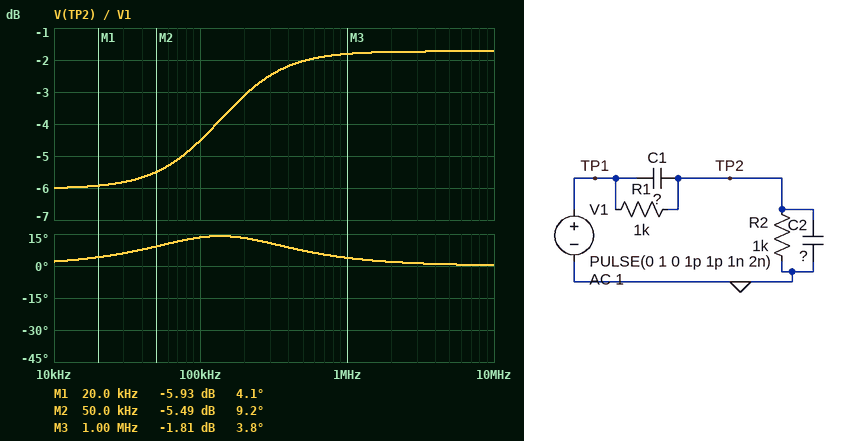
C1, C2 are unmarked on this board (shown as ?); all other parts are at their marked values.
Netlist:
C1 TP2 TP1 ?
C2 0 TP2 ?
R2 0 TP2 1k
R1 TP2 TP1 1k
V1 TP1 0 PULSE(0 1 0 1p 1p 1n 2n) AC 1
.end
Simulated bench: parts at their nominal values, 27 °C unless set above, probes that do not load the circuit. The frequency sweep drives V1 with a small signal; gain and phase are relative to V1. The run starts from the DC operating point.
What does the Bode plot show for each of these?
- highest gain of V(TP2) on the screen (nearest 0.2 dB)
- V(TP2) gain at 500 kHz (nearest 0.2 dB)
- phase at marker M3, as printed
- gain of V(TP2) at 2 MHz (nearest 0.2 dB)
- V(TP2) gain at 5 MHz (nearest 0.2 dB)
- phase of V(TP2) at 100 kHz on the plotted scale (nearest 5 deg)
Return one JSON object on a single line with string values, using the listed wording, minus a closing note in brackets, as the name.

{"highest gain of V(TP2) on the screen": "-1.8 dB", "V(TP2) gain at 500 kHz": "-2.0 dB", "phase at marker M3, as printed": "3.8 deg", "gain of V(TP2) at 2 MHz": "-1.8 dB", "V(TP2) gain at 5 MHz": "-1.8 dB", "phase of V(TP2) at 100 kHz on the plotted scale": "15 deg"}
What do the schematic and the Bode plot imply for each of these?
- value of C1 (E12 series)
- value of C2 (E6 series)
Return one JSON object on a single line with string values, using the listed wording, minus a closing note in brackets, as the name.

{"value of C1": "1.5 nF", "value of C2": "330 pF"}
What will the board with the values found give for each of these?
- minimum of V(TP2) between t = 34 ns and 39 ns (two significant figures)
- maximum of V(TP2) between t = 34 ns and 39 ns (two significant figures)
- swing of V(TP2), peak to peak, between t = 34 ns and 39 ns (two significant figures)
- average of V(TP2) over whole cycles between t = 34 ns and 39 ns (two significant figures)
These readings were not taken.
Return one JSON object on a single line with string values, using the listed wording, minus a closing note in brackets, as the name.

{"minimum of V(TP2) between t = 34 ns and 39 ns": "-6.5 mV", "maximum of V(TP2) between t = 34 ns and 39 ns": "810 mV", "swing of V(TP2), peak to peak, between t = 34 ns and 39 ns": "820 mV", "average of V(TP2) over whole cycles between t = 34 ns and 39 ns": "400 mV"}
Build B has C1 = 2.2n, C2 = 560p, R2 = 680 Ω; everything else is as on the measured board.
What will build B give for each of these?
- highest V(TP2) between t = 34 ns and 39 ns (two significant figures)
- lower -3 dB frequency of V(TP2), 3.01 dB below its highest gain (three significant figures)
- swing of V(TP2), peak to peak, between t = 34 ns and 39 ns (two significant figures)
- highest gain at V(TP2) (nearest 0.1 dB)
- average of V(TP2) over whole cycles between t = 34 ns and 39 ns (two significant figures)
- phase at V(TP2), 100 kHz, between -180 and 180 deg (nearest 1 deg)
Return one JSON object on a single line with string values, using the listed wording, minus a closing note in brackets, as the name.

{"highest V(TP2) between t = 34 ns and 39 ns": "790 mV", "lower -3 dB frequency of V(TP2), 3.01 dB below its highest gain": "99.1 kHz", "swing of V(TP2), peak to peak, between t = 34 ns and 39 ns": "800 mV", "highest gain at V(TP2)": "-2.0 dB", "average of V(TP2) over whole cycles between t = 34 ns and 39 ns": "390 mV", "phase at V(TP2), 100 kHz, between -180 and 180 deg": "19 deg"}
